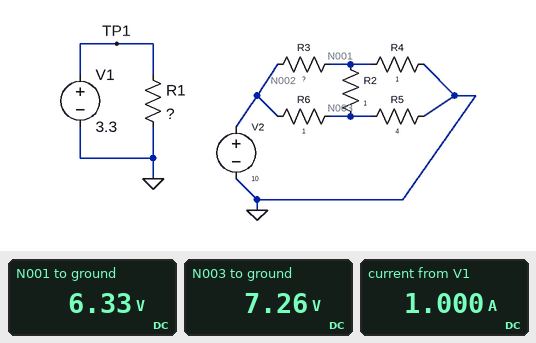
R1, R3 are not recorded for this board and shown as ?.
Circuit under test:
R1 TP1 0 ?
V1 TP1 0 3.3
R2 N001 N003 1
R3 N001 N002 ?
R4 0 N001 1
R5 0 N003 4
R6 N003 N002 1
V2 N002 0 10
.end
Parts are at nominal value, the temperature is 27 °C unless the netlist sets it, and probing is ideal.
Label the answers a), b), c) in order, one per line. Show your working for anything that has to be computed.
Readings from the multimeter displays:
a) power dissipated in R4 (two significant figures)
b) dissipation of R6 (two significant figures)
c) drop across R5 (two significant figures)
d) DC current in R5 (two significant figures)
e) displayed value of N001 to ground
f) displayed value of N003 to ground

a) (6.33 V)^2 / 1 Ω = 40 W
b) (10 V - 7.26 V)^2 / 1 Ω = 7.5 W
c) 7.26 V = 7.3 V
d) (7.26 V) / 4 Ω = 1.8 A
e) 6.33 V
f) 7.26 V
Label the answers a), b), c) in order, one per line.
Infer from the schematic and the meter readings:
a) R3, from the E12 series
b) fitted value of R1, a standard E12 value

a) 0.68 Ω
b) 3.3 Ω
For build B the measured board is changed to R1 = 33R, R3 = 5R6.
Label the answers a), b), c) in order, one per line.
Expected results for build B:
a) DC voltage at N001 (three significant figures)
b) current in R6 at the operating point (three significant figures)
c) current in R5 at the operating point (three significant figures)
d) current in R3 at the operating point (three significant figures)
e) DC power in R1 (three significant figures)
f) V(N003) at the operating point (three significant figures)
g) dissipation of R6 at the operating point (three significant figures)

a) 3.59 V
b) 3.96 A
c) 1.51 A
d) 1.14 A
e) 330 mW
f) 6.04 V
g) 15.7 W
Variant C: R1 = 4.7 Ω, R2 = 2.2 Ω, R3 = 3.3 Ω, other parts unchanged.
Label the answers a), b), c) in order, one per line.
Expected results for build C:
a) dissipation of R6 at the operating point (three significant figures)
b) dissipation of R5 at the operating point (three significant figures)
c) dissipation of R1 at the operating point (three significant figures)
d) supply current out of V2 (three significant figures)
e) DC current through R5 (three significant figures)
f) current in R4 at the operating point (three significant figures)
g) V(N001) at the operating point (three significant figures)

a) 10.3 W
b) 11.5 W
c) 2.32 W
d) 5.18 A
e) 1.70 A
f) 3.48 A
g) 3.48 V
